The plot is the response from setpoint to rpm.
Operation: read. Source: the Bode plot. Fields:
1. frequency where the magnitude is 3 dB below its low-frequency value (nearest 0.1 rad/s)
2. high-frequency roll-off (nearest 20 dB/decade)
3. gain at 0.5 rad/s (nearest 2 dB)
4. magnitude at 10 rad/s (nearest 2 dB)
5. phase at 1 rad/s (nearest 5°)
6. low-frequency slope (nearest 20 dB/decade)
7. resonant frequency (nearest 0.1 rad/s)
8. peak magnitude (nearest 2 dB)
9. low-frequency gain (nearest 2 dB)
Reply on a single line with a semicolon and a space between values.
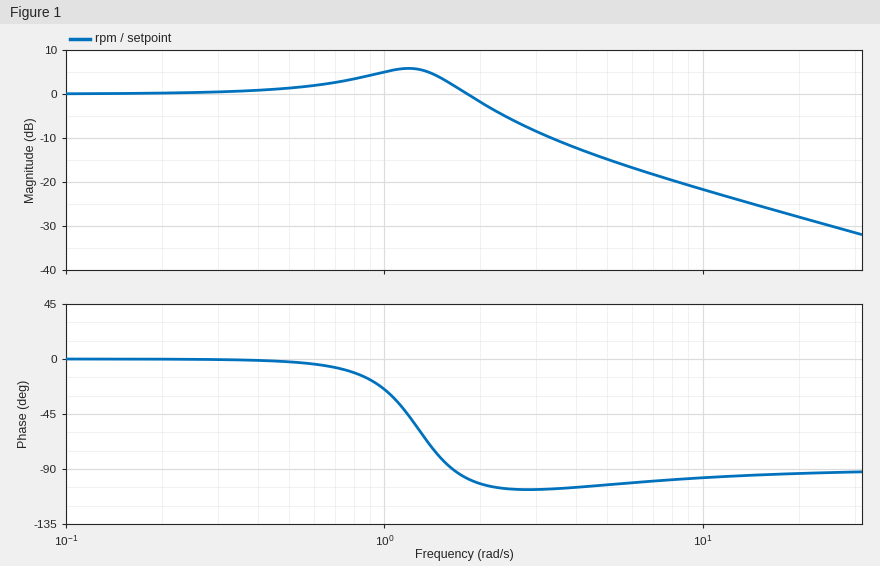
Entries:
2.1 rad/s; -20 dB/decade; 2 dB; -22 dB; -25°; 0 dB/decade; 1.2 rad/s; 6 dB; 0 dB
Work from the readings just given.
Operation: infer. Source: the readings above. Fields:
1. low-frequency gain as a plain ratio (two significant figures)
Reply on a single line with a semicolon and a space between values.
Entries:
1.0
